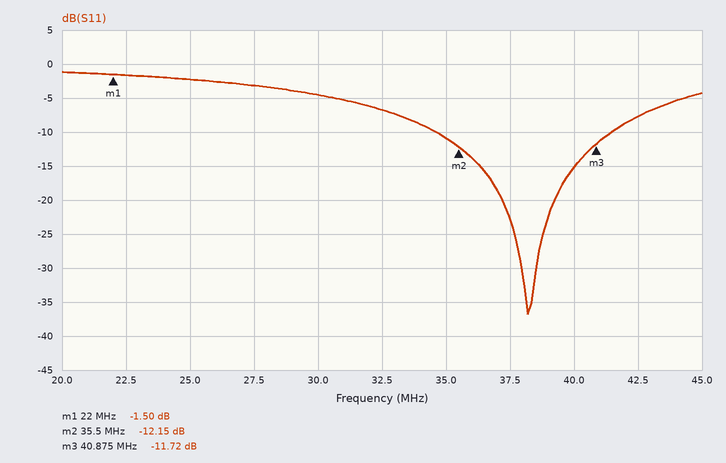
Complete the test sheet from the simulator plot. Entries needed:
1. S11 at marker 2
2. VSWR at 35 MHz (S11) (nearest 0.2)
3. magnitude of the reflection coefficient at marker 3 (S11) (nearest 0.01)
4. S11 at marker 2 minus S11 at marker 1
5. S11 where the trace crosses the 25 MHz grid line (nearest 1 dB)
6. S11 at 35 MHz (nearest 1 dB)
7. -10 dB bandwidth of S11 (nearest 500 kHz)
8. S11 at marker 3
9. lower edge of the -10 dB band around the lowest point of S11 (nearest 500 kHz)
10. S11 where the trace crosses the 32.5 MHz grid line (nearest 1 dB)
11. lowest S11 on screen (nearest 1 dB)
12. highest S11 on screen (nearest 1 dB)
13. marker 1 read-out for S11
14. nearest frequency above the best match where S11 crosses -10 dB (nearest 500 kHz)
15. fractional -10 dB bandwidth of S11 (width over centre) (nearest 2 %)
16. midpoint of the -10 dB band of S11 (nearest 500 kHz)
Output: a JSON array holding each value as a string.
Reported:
["-12.15 dB", "1.8", "0.26", "-10.65 dB", "-2 dB", "-11 dB", "7.0 MHz", "-11.72 dB", "34.5 MHz", "-7 dB", "-37 dB", "-1 dB", "-1.50 dB", "41.5 MHz", "18 %", "38.0 MHz"]
